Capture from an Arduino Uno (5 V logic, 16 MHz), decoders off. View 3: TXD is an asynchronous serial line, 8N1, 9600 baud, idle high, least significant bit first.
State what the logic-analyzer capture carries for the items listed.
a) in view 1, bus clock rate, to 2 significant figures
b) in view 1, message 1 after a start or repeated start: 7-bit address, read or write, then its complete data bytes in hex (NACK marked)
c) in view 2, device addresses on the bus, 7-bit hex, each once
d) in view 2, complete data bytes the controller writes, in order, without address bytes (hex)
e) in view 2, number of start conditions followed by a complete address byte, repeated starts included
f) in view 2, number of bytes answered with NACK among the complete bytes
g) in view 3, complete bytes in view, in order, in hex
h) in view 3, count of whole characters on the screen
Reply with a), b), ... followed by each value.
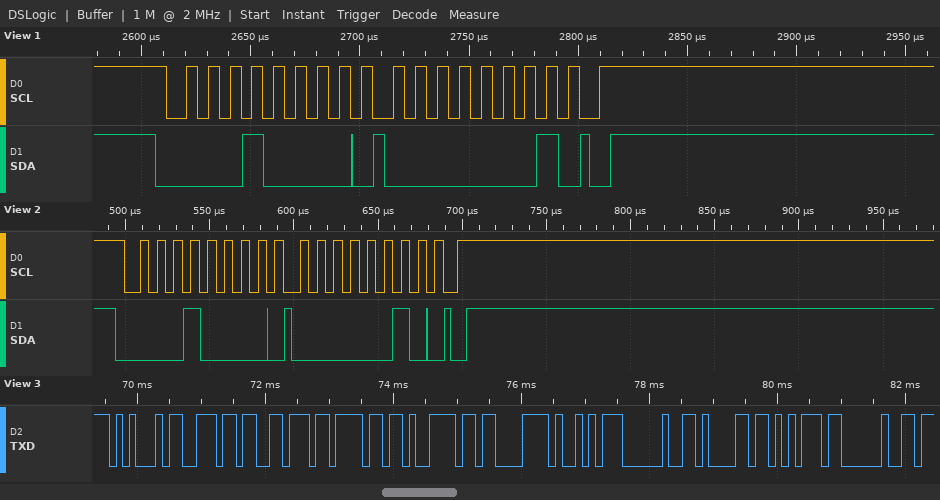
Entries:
a) 100 kHz
b) 0x08 write: 01
c) 0x08
d) 02
e) 1
f) 0
g) 0x45 0x6E 0x76 0x6F 0x79 0xC3 0xA9 0x20 0x61 0x75 0x20
h) 11
